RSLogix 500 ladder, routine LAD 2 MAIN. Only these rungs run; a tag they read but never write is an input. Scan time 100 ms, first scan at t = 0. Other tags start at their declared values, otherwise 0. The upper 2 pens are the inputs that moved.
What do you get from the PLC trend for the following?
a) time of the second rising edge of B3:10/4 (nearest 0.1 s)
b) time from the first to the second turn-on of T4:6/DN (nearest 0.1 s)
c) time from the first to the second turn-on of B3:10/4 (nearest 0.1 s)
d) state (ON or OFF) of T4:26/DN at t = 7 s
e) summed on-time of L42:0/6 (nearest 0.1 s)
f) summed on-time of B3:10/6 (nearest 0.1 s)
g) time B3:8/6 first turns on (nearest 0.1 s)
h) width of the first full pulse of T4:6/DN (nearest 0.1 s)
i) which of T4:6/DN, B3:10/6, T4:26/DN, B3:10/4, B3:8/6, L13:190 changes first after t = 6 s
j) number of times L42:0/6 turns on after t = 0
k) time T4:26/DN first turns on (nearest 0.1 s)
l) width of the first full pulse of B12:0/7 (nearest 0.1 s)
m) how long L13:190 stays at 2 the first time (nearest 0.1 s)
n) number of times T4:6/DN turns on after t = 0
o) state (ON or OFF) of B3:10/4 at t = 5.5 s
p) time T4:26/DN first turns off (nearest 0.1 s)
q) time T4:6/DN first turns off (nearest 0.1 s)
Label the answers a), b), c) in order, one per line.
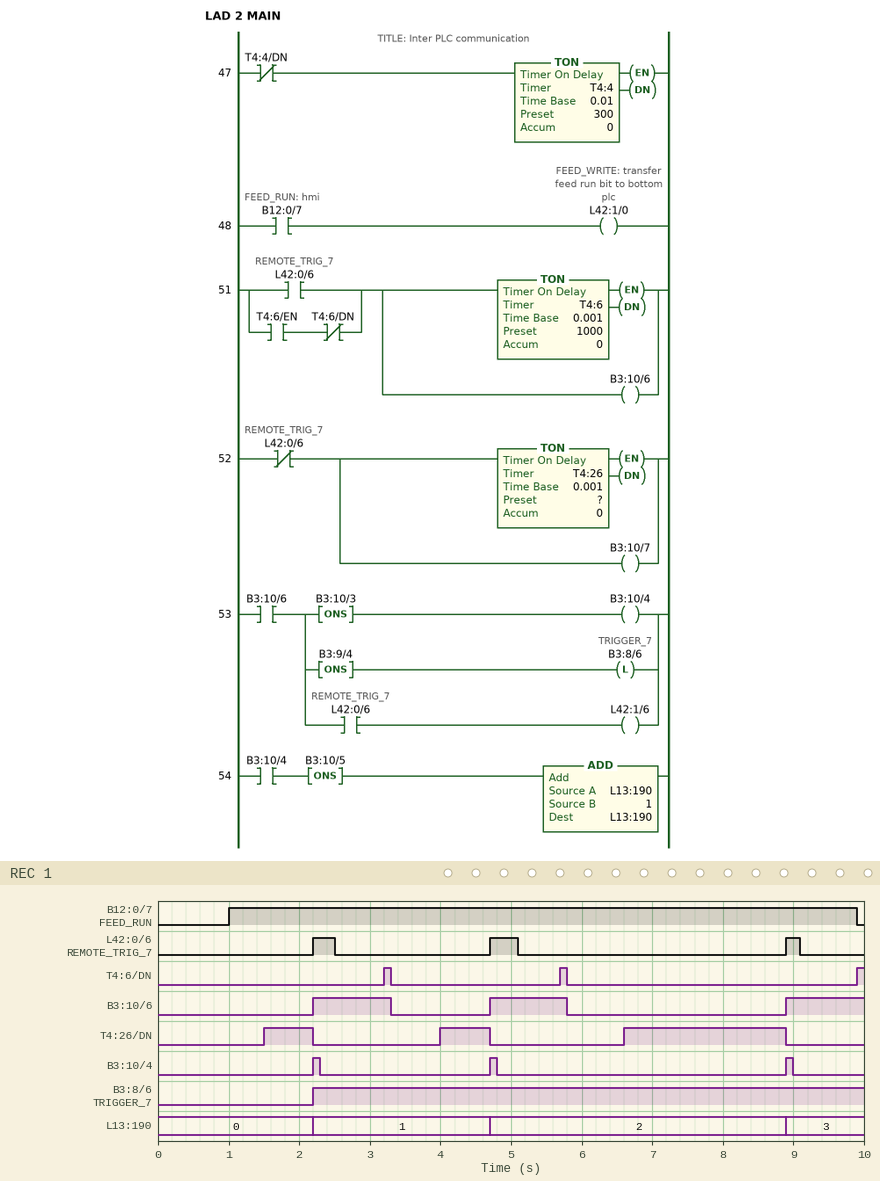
a) 4.7 s
b) 2.5 s
c) 2.5 s
d) ON
e) 0.9 s
f) 3.3 s
g) 2.2 s
h) 0.1 s
i) T4:26/DN
j) 3
k) 1.5 s
l) 8.9 s
m) 4.2 s
n) 3
o) OFF
p) 2.2 s
q) 3.3 s
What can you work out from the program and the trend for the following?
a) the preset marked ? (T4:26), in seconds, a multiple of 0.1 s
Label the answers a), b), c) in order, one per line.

a) 1.5 s
